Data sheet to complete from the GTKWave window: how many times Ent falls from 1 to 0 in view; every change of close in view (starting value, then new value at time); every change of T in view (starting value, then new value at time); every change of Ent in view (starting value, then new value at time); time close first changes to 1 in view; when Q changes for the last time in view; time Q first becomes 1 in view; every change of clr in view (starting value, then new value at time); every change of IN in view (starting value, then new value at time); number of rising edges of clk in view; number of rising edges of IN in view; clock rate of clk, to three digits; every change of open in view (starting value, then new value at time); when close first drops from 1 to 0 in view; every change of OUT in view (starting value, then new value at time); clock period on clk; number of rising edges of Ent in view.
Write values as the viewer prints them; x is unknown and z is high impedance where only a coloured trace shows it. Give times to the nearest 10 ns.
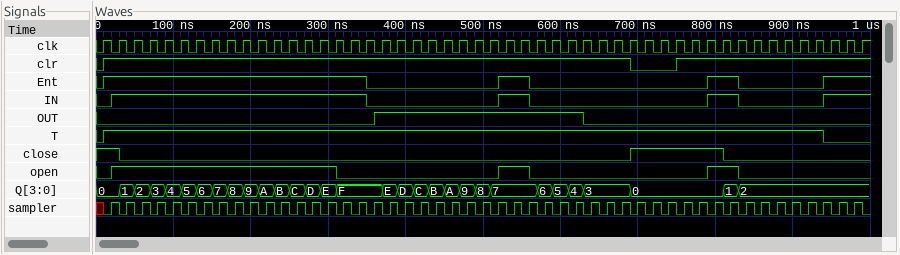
3
1, 0 at 30 ns, 1 at 690 ns, 0 at 810 ns
0, 1 at 10 ns, 0 at 940 ns
0, 1 at 10 ns, 0 at 350 ns, 1 at 520 ns, 0 at 560 ns, 1 at 790 ns, 0 at 830 ns, 1 at 940 ns
690 ns
830 ns
30 ns
0, 1 at 10 ns, 0 at 690 ns, 1 at 750 ns
0, 1 at 20 ns, 0 at 350 ns, 1 at 520 ns, 0 at 560 ns, 1 at 790 ns, 0 at 830 ns, 1 at 940 ns
50
4
50.0 MHz
0, 1 at 20 ns, 0 at 310 ns, 1 at 520 ns, 0 at 560 ns, 1 at 790 ns, 0 at 830 ns
30 ns
0, 1 at 360 ns, 0 at 630 ns
20 ns
4
